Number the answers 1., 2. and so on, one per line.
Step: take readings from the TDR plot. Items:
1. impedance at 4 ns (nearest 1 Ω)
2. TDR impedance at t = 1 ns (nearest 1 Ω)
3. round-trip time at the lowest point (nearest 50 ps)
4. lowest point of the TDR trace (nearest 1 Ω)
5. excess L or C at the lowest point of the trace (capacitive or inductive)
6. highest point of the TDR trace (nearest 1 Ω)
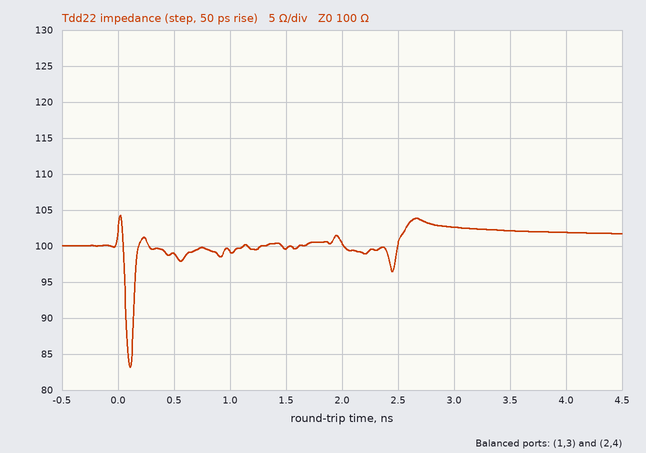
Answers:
1. 102 Ω
2. 99 Ω
3. 100 ps
4. 83 Ω
5. capacitive
6. 104 Ω
